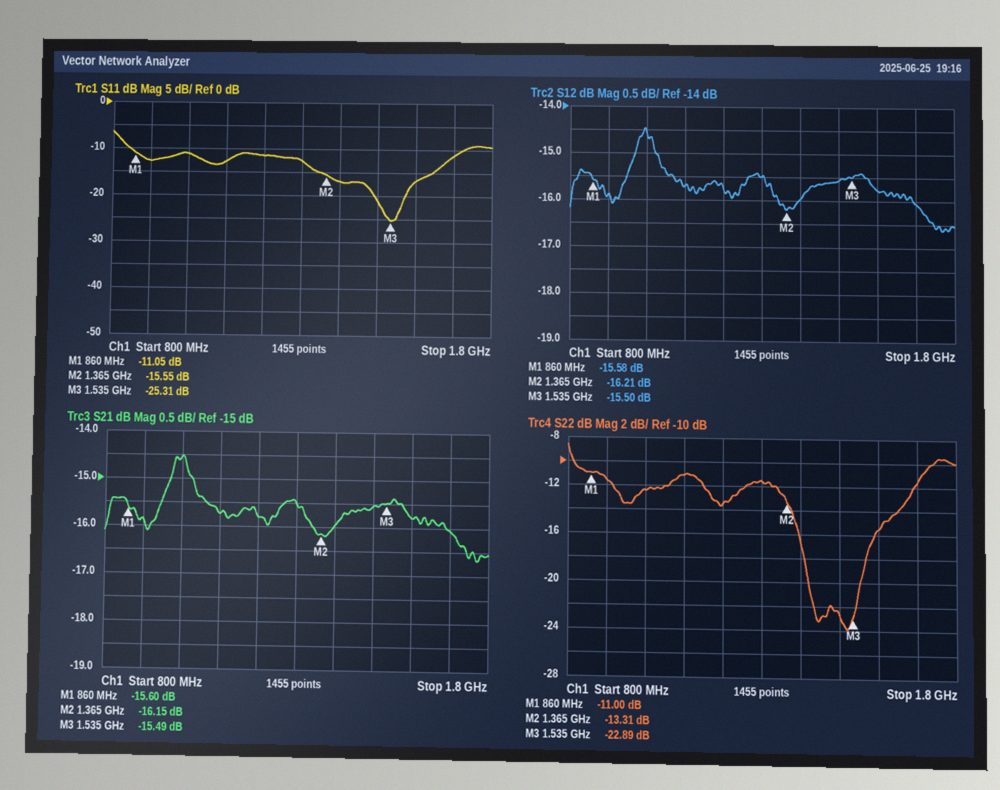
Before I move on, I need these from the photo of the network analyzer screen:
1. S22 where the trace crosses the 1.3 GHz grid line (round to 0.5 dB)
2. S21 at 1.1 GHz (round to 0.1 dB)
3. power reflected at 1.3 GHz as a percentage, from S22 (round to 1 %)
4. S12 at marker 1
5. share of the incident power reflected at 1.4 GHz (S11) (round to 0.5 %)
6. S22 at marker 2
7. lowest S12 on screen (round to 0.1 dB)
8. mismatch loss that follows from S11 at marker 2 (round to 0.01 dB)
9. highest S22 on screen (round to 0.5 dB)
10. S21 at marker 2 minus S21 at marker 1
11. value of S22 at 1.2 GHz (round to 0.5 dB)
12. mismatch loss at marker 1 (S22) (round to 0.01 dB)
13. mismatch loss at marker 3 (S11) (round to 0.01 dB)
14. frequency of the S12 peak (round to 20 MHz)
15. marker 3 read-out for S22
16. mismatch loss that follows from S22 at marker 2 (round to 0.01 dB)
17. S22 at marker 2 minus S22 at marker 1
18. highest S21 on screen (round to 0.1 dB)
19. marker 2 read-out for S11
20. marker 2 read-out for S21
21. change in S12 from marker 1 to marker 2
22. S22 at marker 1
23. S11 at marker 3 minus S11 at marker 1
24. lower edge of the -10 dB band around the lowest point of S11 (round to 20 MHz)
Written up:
-11.5 dB
-15.7 dB
7 %
-15.58 dB
2.0 %
-13.31 dB
-16.6 dB
0.12 dB
-8.5 dB
-0.55 dB
-13.5 dB
0.36 dB
0.01 dB
1.00 GHz
-22.89 dB
0.21 dB
-2.31 dB
-14.5 dB
-15.55 dB
-16.15 dB
-0.63 dB
-11.00 dB
-14.26 dB
840 MHz
